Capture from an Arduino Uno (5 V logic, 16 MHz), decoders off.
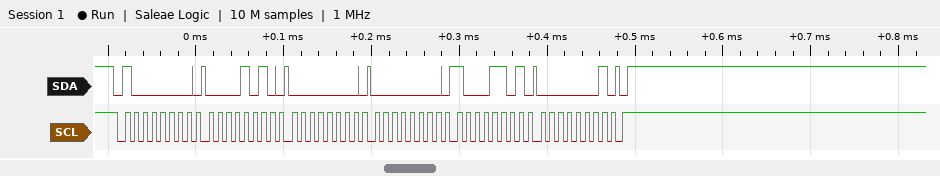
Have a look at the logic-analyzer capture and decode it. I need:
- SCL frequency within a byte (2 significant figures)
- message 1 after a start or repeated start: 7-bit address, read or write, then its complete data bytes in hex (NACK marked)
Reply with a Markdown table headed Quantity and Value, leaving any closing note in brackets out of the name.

| Quantity | Value |
|---|---|
| SCL frequency within a byte | 100 kHz |
| message 1 after a start or repeated start: 7-bit address, read or write, then its complete data bytes in hex | 0x40 write: 0A 00 00 8D 01 |
